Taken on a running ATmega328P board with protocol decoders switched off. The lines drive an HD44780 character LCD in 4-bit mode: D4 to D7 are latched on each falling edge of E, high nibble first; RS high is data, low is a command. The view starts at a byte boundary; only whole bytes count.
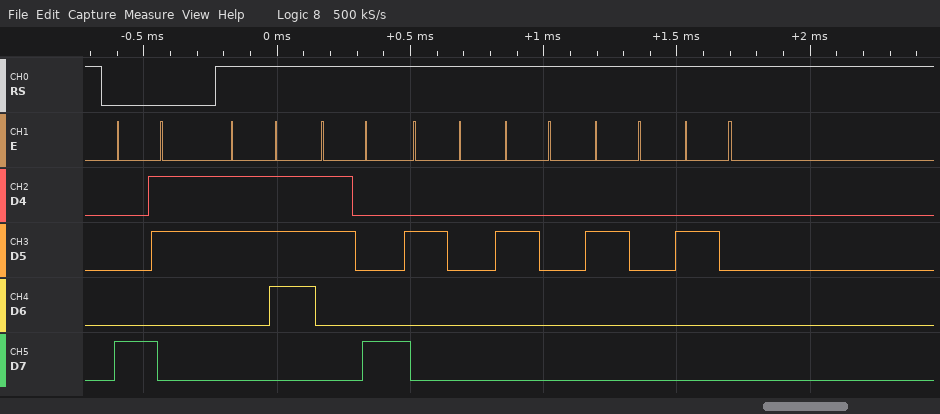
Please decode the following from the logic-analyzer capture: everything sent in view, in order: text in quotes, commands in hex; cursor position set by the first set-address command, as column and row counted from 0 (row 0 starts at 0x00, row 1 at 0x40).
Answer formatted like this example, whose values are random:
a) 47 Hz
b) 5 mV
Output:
a) 0x83 "78    "
b) column 3, row 0
